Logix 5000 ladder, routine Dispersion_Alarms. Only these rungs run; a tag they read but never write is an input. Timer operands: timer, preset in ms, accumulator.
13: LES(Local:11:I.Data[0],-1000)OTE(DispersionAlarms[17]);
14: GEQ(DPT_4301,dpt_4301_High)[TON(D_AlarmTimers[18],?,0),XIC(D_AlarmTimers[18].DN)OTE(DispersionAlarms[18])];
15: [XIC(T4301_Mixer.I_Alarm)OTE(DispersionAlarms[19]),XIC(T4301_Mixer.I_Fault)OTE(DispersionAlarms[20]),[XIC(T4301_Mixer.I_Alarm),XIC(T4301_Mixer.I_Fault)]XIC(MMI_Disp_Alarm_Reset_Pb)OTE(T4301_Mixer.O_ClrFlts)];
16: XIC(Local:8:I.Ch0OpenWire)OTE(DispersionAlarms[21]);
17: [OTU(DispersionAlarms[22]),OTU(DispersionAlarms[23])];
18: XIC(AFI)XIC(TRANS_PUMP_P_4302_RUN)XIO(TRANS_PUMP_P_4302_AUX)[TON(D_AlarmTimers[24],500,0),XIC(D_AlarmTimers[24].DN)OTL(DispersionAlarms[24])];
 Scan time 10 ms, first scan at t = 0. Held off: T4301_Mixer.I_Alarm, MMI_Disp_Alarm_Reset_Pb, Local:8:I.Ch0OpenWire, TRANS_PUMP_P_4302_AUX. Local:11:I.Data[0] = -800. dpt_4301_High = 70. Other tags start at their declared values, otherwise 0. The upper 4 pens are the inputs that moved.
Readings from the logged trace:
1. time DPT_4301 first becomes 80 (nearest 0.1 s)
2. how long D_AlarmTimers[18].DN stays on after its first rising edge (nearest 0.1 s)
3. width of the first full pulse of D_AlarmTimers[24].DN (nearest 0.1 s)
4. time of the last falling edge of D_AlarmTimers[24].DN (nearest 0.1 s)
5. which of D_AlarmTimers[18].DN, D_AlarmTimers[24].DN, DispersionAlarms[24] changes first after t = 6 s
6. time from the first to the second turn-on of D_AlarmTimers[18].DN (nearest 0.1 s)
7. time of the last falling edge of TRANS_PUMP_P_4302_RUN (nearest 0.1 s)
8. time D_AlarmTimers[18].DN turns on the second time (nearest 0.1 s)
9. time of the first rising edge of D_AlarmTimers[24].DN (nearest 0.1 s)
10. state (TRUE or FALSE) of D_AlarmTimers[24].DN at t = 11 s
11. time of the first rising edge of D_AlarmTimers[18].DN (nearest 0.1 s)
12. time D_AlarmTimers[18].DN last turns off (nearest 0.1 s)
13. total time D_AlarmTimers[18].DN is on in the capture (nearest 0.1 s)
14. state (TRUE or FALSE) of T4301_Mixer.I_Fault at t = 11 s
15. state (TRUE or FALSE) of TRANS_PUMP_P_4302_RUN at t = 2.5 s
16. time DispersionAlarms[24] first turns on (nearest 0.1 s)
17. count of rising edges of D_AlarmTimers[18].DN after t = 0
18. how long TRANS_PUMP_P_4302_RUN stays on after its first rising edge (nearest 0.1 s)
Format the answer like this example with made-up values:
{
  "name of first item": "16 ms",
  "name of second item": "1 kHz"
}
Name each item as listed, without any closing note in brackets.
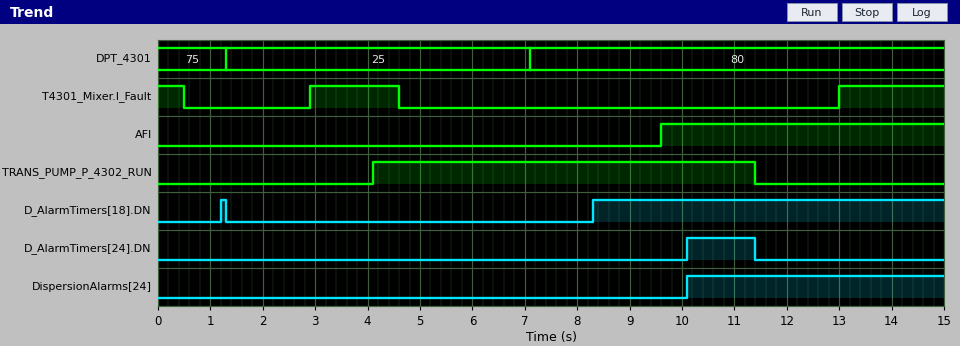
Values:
{
  "time DPT_4301 first becomes 80": "7.1 s",
  "how long D_AlarmTimers[18].DN stays on after its first rising edge": "0.1 s",
  "width of the first full pulse of D_AlarmTimers[24].DN": "1.3 s",
  "time of the last falling edge of D_AlarmTimers[24].DN": "11.4 s",
  "which of D_AlarmTimers[18].DN, D_AlarmTimers[24].DN, DispersionAlarms[24] changes first after t = 6 s": "D_AlarmTimers[18].DN",
  "time from the first to the second turn-on of D_AlarmTimers[18].DN": "7.1 s",
  "time of the last falling edge of TRANS_PUMP_P_4302_RUN": "11.4 s",
  "time D_AlarmTimers[18].DN turns on the second time": "8.3 s",
  "time of the first rising edge of D_AlarmTimers[24].DN": "10.1 s",
  "state (TRUE or FALSE) of D_AlarmTimers[24].DN at t = 11 s": "TRUE",
  "time of the first rising edge of D_AlarmTimers[18].DN": "1.2 s",
  "time D_AlarmTimers[18].DN last turns off": "1.3 s",
  "total time D_AlarmTimers[18].DN is on in the capture": "6.8 s",
  "state (TRUE or FALSE) of T4301_Mixer.I_Fault at t = 11 s": "FALSE",
  "state (TRUE or FALSE) of TRANS_PUMP_P_4302_RUN at t = 2.5 s": "FALSE",
  "time DispersionAlarms[24] first turns on": "10.1 s",
  "count of rising edges of D_AlarmTimers[18].DN after t = 0": "2",
  "how long TRANS_PUMP_P_4302_RUN stays on after its first rising edge": "7.3 s"
}
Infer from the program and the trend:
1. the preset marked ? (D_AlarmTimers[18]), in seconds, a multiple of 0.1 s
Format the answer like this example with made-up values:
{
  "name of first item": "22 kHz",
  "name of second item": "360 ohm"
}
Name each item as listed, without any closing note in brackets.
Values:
{
  "the preset marked ? (D_AlarmTimers[18]), in seconds, a multiple of 0.1 s": "1.2 s"
}
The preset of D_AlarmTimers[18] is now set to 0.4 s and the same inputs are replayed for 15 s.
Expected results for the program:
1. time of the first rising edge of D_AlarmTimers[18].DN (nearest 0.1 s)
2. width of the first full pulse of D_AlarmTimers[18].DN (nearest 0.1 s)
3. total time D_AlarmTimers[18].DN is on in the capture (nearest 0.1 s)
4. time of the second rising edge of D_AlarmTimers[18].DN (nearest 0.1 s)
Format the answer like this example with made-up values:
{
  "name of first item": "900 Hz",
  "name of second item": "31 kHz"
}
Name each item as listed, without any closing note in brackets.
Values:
{
  "time of the first rising edge of D_AlarmTimers[18].DN": "0.4 s",
  "width of the first full pulse of D_AlarmTimers[18].DN": "0.9 s",
  "total time D_AlarmTimers[18].DN is on in the capture": "8.4 s",
  "time of the second rising edge of D_AlarmTimers[18].DN": "7.5 s"
}
